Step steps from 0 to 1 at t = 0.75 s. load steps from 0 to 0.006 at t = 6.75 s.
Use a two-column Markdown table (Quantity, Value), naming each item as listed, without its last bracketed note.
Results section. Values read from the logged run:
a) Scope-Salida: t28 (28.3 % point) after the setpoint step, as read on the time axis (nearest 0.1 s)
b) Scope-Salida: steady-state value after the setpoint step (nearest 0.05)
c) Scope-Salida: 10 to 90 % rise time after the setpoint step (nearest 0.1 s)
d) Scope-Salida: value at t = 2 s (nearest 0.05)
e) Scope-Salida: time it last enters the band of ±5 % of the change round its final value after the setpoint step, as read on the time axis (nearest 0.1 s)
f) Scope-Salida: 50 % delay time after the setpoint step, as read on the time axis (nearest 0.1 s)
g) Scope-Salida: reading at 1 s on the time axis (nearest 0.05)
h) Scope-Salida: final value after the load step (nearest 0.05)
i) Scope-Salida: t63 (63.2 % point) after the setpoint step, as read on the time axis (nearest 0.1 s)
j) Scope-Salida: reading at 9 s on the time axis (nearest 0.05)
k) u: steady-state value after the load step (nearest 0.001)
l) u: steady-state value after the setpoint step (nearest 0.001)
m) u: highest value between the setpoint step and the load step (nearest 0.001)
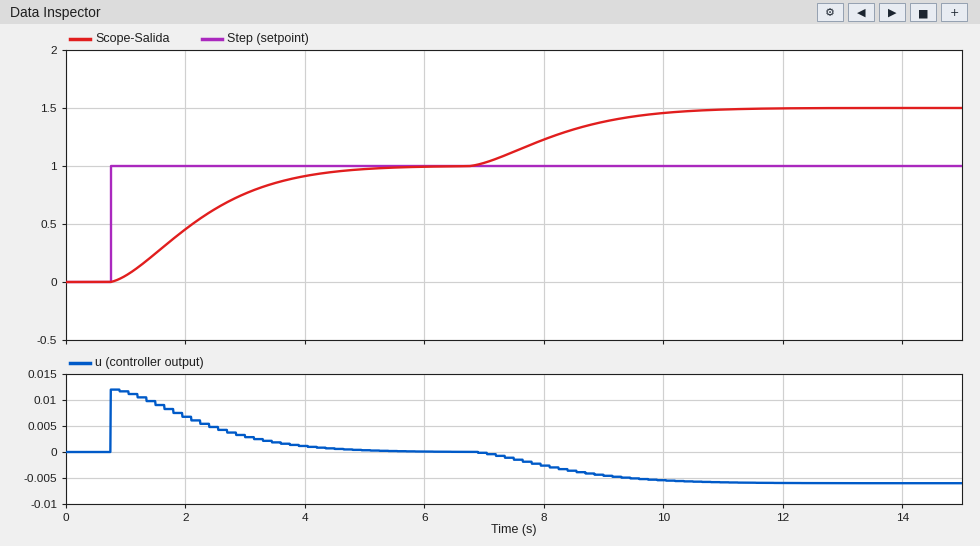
| Quantity | Value |
|---|---|
| Scope-Salida: t28 (28.3 % point) after the setpoint step, as read on the time axis | 1.6 s |
| Scope-Salida: steady-state value after the setpoint step | 1.00 |
| Scope-Salida: 10 to 90 % rise time after the setpoint step | 2.7 s |
| Scope-Salida: value at t = 2 s | 0.45 |
| Scope-Salida: time it last enters the band of ±5 % of the change round its final value after the setpoint step, as read on the time axis | 4.5 s |
| Scope-Salida: 50 % delay time after the setpoint step, as read on the time axis | 2.1 s |
| Scope-Salida: reading at 1 s on the time axis | 0.05 |
| Scope-Salida: final value after the load step | 1.50 |
| Scope-Salida: t63 (63.2 % point) after the setpoint step, as read on the time axis | 2.5 s |
| Scope-Salida: reading at 9 s on the time axis | 1.40 |
| u: steady-state value after the load step | -0.006 |
| u: steady-state value after the setpoint step | 0.000 |
| u: highest value between the setpoint step and the load step | 0.012 |
